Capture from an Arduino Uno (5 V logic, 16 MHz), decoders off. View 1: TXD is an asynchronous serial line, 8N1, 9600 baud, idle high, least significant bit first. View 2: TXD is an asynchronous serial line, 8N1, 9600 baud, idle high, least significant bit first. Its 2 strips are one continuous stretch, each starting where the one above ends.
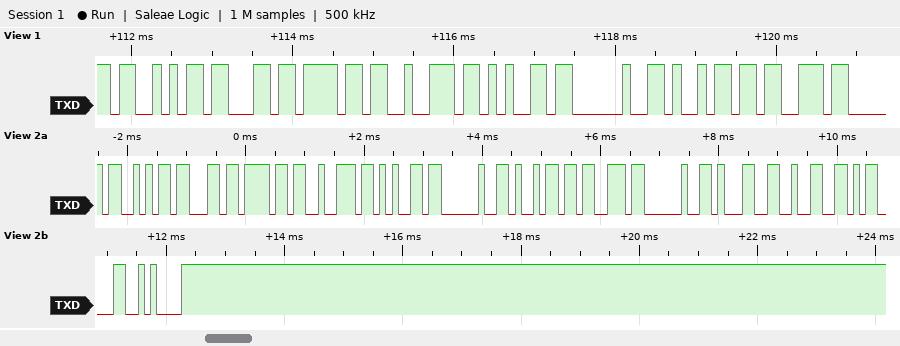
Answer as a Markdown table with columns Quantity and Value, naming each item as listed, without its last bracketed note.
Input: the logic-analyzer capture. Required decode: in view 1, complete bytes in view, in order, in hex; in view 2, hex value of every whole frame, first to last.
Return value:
| Quantity | Value |
|---|---|
| in view 1, complete bytes in view, in order, in hex | 0x53 0x63 0x6F 0x72 0x65 0x20 0x69 0x73 |
| in view 2, hex value of every whole frame, first to last | 53 63 6F 72 65 20 69 73 20 31 32 0D 0A |
